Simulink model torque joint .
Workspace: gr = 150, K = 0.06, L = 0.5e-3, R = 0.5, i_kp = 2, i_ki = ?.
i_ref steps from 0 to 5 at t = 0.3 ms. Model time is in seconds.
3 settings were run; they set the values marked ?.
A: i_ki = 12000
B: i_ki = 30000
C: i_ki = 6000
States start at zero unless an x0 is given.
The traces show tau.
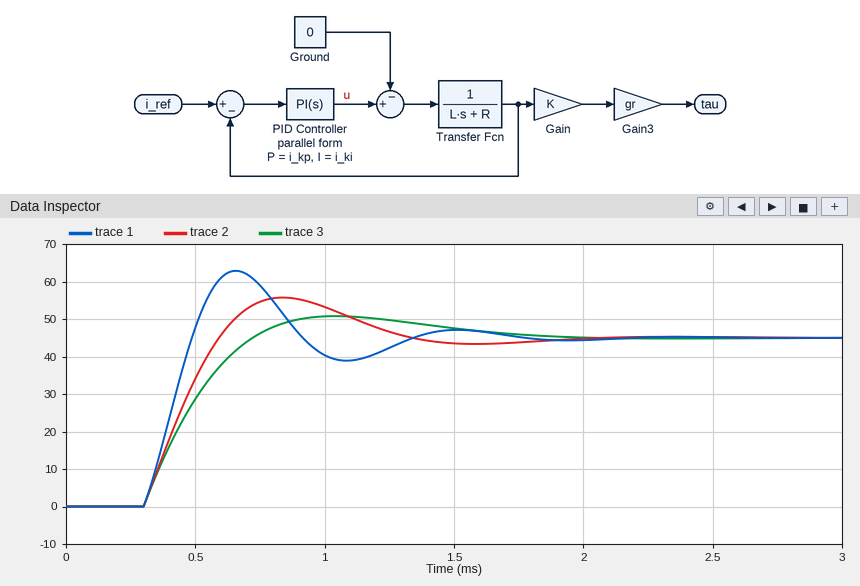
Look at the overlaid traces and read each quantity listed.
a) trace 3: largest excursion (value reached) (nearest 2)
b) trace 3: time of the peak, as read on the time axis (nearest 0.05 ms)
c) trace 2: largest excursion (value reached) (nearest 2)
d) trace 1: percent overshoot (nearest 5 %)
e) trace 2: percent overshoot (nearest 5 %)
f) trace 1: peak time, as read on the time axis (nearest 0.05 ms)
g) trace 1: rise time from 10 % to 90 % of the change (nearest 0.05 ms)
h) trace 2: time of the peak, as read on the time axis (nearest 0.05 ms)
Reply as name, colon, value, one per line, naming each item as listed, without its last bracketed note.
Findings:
trace 3: largest excursion (value reached): 50
trace 3: time of the peak, as read on the time axis: 1.05 ms
trace 2: largest excursion (value reached): 56
trace 1: percent overshoot: 40 %
trace 2: percent overshoot: 25 %
trace 1: peak time, as read on the time axis: 0.65 ms
trace 1: rise time from 10 % to 90 % of the change: 0.15 ms
trace 2: time of the peak, as read on the time axis: 0.85 ms
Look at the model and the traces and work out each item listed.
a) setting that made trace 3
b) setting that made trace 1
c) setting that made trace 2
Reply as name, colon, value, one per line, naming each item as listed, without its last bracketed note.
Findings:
setting that made trace 3: C
setting that made trace 1: B
setting that made trace 2: A
